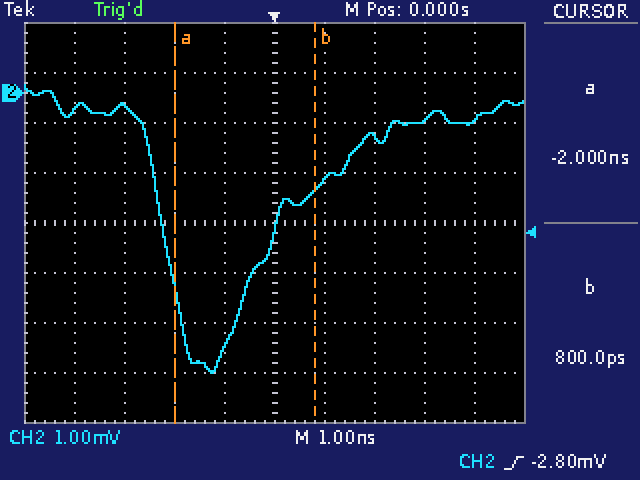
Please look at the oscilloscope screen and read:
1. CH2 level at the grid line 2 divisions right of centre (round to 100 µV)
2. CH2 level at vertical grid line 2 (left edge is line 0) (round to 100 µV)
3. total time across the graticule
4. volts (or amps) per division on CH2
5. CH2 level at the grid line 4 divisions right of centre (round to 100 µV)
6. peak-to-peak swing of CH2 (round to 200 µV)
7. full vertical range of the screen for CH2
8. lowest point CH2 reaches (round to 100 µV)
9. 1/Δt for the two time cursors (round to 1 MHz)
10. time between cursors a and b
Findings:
-900 µV
-300 µV
10 ns
1 mV
-500 µV
5.8 mV
8 mV
-5.6 mV
357 MHz
2.8 ns
